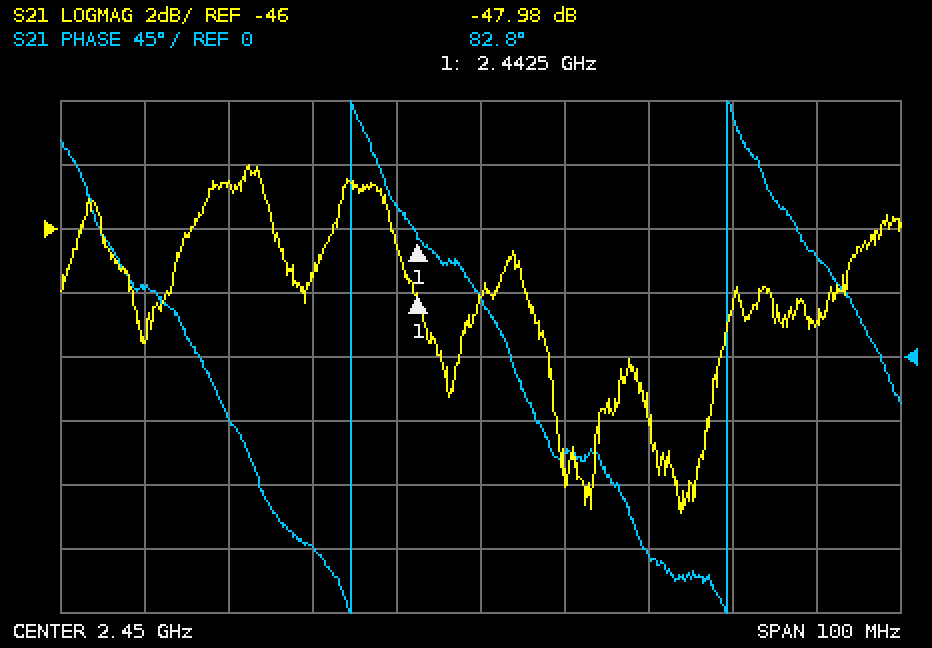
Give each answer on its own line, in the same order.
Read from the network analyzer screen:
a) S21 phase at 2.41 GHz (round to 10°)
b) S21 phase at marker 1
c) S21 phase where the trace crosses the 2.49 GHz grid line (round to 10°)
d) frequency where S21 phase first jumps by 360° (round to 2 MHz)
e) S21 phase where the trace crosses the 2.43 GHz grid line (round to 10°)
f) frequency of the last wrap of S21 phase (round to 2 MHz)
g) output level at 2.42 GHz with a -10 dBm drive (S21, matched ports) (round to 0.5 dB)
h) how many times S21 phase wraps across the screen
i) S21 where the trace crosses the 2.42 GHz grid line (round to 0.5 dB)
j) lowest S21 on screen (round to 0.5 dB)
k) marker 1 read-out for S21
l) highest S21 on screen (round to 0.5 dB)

50°
82.8°
70°
2.434 GHz
-130°
2.480 GHz
-54.5 dBm
2
-44.5 dB
-55.0 dB
-47.98 dB
-44.0 dB
